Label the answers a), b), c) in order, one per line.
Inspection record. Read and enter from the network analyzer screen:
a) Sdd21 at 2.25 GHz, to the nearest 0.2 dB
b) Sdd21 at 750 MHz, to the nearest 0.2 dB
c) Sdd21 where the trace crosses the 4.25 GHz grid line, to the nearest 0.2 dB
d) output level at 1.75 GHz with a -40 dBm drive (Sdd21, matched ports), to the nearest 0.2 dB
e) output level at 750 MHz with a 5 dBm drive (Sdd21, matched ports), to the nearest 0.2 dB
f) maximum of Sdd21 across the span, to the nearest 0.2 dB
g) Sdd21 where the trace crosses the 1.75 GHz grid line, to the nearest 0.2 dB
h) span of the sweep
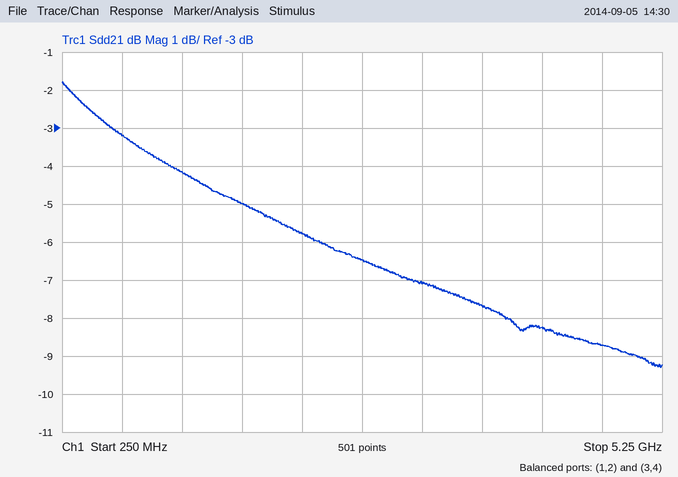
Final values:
a) -5.8 dB
b) -3.2 dB
c) -8.2 dB
d) -45.0 dBm
e) 1.8 dBm
f) -1.8 dB
g) -5.0 dB
h) 5 GHz
